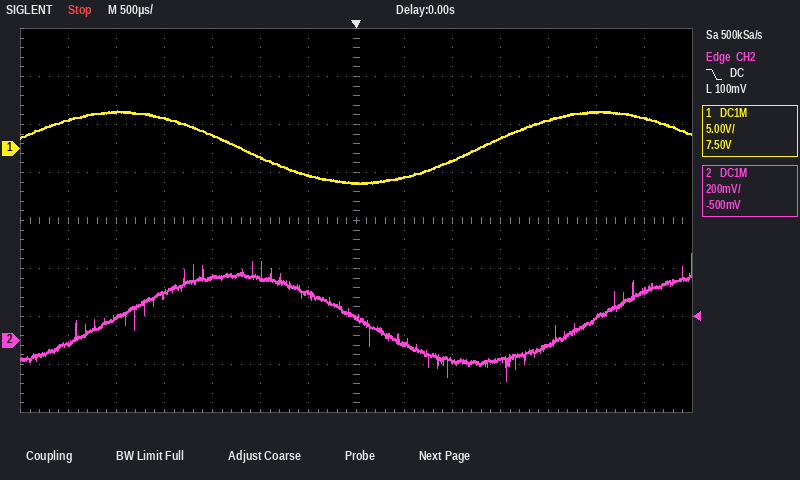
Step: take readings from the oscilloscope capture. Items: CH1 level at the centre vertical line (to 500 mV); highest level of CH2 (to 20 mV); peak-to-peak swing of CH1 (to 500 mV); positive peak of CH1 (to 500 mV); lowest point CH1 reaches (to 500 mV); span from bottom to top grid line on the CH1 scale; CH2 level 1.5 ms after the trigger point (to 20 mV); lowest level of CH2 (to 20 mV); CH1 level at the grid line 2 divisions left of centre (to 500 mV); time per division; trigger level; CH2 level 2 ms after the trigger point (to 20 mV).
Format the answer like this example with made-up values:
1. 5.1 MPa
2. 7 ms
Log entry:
1. -3.5 V
2. 360 mV
3. 7.5 V
4. 4.0 V
5. -3.5 V
6. 40 V
7. -80 mV
8. -160 mV
9. -1.0 V
10. 500 µs
11. 100 mV
12. -20 mV
